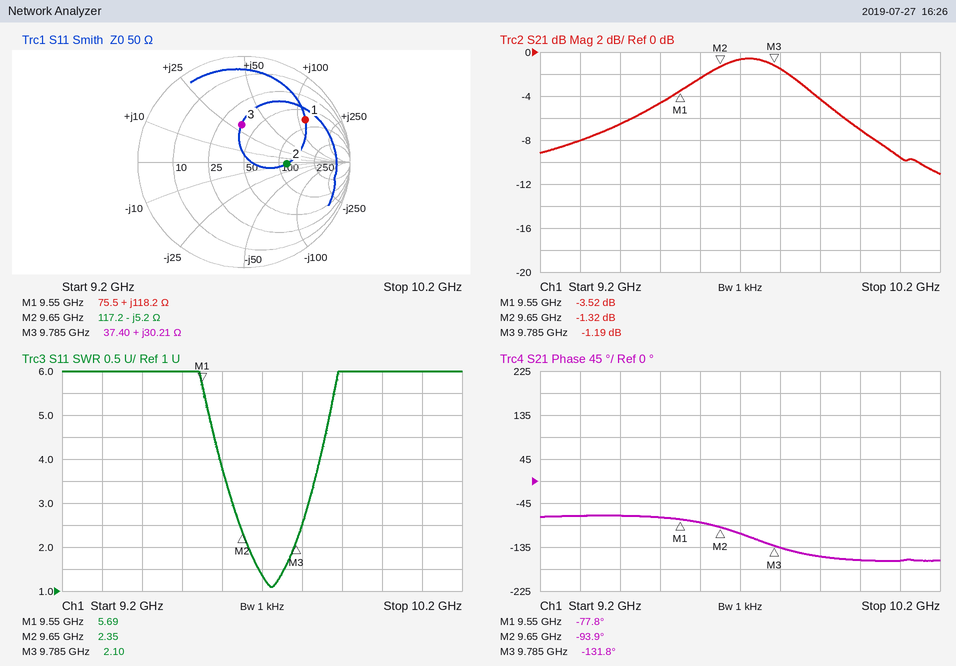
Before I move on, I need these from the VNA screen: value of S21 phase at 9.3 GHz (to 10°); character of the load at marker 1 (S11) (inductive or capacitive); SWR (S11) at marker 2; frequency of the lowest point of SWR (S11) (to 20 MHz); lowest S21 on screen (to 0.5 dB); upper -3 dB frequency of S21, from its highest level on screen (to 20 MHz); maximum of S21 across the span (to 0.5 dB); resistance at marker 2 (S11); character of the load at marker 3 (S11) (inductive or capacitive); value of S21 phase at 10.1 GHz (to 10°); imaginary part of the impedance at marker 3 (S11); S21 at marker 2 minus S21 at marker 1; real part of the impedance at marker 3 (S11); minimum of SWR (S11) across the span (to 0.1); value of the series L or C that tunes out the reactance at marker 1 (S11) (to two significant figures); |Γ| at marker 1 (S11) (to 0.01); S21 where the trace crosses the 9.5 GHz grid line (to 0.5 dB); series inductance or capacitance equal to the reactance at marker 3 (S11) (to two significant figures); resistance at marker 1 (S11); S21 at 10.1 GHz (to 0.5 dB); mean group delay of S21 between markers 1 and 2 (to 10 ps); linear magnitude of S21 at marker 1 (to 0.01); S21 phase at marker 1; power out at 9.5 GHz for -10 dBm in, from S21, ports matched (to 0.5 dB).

-70°
inductive
2.35
9.72 GHz
-11.0 dB
9.88 GHz
-0.5 dB
117.2 Ω
inductive
-160°
+30.21 Ω
2.20 dB
37.40 Ω
1.1
140 fF
0.70
-4.5 dB
490 pH
75.5 Ω
-9.5 dB
450 ps
0.67
-77.8°
-14.5 dBm
